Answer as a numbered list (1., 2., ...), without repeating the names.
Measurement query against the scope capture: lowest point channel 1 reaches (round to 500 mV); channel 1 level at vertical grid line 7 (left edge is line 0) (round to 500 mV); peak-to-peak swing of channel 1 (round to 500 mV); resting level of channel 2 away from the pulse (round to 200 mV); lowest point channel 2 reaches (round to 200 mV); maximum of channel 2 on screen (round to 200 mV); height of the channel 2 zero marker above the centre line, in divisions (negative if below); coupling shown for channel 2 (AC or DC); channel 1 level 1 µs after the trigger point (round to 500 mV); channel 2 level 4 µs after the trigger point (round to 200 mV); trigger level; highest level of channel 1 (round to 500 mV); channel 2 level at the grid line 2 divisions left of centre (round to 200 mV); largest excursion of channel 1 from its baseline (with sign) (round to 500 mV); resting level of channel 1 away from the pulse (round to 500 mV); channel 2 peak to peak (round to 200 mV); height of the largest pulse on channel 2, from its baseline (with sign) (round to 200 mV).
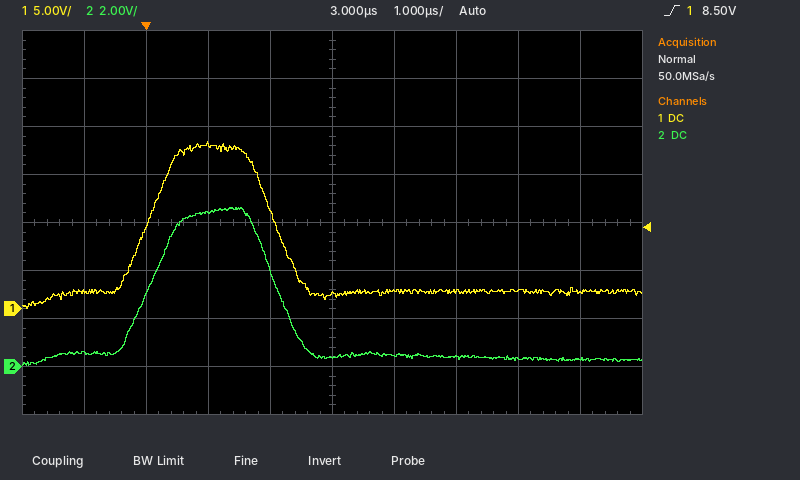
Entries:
1. 0.0 V
2. 2.0 V
3. 17.5 V
4. 400 mV
5. 0.0 V
6. 6.6 V
7. -3.0 div
8. DC
9. 17.0 V
10. 400 mV
11. 8.50 V
12. 17.5 V
13. 6.4 V
14. +15.5 V
15. 2.0 V
16. 6.6 V
17. +6.2 V
